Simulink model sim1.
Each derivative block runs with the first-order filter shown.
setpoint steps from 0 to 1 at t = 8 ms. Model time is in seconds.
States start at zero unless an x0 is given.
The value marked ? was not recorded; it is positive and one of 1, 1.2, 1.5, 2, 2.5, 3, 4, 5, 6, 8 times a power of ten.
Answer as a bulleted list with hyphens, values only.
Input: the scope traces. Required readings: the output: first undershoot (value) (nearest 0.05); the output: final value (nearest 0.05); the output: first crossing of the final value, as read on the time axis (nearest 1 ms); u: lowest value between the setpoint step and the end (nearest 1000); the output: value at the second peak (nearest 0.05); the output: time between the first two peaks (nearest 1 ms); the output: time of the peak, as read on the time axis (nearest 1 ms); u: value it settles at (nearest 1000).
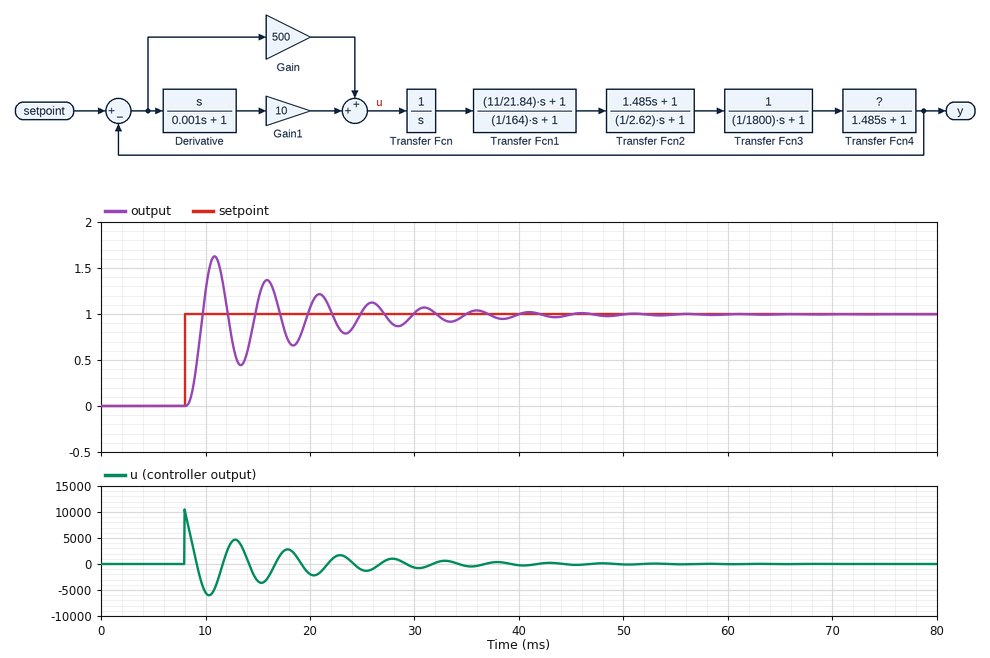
- 0.45
- 1.00
- 10 ms
- -6000
- 1.35
- 5 ms
- 11 ms
- 0
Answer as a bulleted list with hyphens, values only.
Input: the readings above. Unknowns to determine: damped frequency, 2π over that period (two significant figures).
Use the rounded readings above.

- 1.3 rad/ms
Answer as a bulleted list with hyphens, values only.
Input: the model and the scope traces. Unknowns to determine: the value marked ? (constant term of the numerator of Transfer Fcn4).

- 1
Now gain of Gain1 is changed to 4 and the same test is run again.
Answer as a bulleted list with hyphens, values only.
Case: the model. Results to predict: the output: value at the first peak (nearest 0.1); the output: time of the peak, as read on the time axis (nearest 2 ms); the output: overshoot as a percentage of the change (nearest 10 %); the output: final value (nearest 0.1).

- 1.3
- 12 ms
- 30 %
- 1.0
